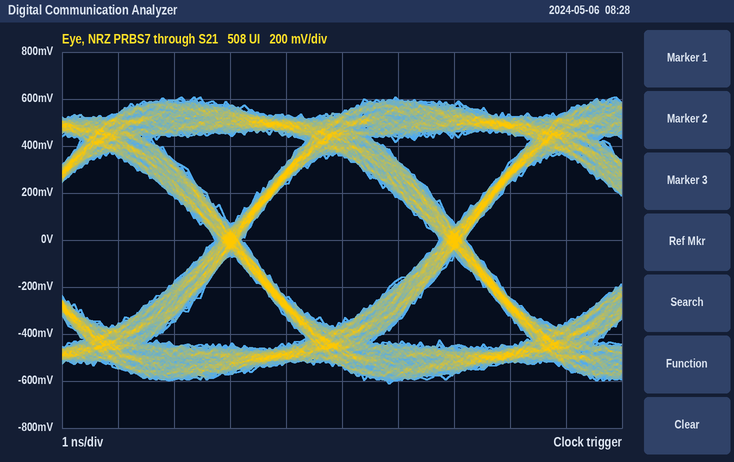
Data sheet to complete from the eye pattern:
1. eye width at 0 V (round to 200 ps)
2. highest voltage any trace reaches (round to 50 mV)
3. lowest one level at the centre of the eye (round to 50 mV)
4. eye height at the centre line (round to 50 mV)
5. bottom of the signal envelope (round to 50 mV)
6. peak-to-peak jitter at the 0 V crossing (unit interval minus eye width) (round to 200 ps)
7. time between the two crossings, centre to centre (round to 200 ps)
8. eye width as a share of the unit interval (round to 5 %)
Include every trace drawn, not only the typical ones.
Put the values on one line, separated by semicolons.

3.6 ns; 600 mV; 350 mV; 700 mV; -600 mV; 400 ps; 4.0 ns; 90 %
